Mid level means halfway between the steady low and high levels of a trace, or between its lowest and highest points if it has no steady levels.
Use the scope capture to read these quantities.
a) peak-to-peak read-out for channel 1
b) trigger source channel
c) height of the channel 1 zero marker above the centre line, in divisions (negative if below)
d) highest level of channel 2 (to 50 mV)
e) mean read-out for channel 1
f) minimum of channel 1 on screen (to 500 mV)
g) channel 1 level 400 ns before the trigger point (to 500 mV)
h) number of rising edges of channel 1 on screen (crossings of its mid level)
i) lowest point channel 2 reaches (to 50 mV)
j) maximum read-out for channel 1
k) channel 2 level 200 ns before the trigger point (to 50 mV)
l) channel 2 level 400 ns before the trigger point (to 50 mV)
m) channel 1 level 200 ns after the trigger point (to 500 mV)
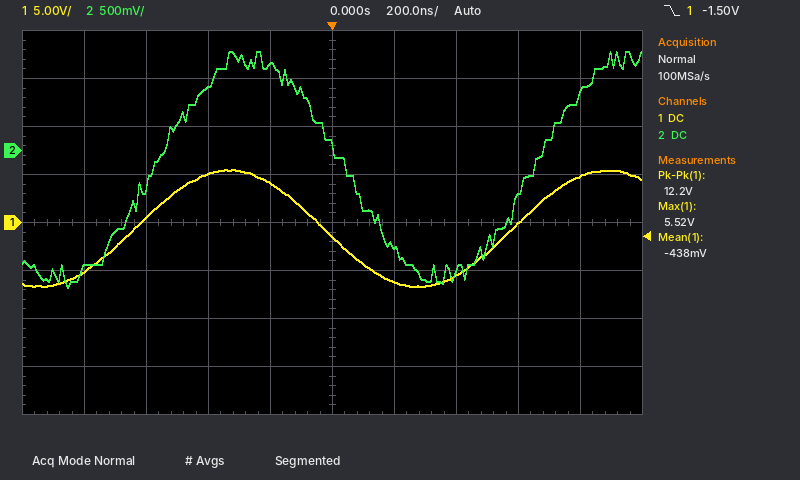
12.2 V
channel 1
0.0 div
1.05 V
-438 mV
-6.5 V
5.0 V
2
-1.45 V
5.52 V
900 mV
650 mV
-6.0 V
